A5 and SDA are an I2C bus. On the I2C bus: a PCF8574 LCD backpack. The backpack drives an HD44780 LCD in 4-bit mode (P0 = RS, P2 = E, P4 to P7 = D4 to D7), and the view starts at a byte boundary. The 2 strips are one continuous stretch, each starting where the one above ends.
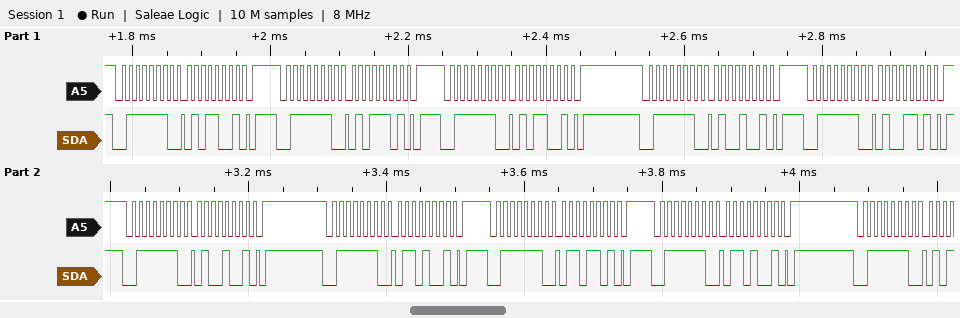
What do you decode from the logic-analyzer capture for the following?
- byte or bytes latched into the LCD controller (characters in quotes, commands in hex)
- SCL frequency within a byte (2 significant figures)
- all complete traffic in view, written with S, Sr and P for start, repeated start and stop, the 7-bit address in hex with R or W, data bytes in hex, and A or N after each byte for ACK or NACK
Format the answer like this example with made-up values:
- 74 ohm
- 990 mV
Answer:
- 'T'
- 100 kHz
- S 3FW A 59 A P S 3FW A 5D A P S 3FW A 59 A P S 3FW A 49 A P S 3FW A 4D A P S 3FW A 49 A P S 3FW A 69 A P S 3FW A 6D A P S 3FW A 69 A P S 3FW A
